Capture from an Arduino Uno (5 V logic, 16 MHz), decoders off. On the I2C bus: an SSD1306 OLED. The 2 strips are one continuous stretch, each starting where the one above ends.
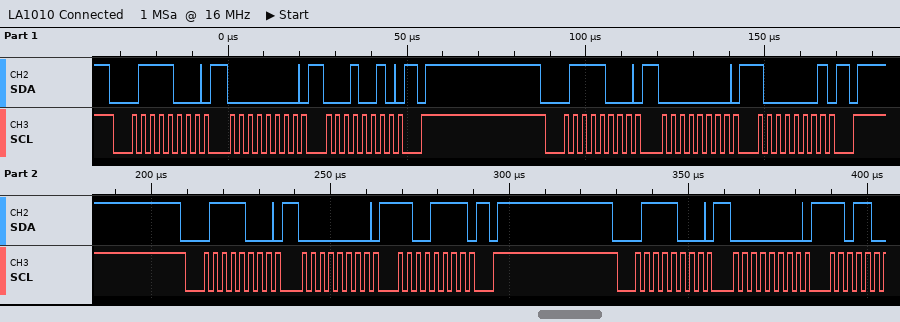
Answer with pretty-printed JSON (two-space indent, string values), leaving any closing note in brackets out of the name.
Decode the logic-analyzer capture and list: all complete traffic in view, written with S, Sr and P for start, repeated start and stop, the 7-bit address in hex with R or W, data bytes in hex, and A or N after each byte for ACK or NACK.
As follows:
{
  "all complete traffic in view, written with S, Sr and P for start, repeated start and stop, the 7-bit address in hex with R or W, data bytes in hex, and A or N after each byte for ACK or NACK": "S 3CW A 00 A 12 A P S 3CW A 00 A 81 A P S 3CW A 00 A CF A P S 3CW A 00 A"
}
